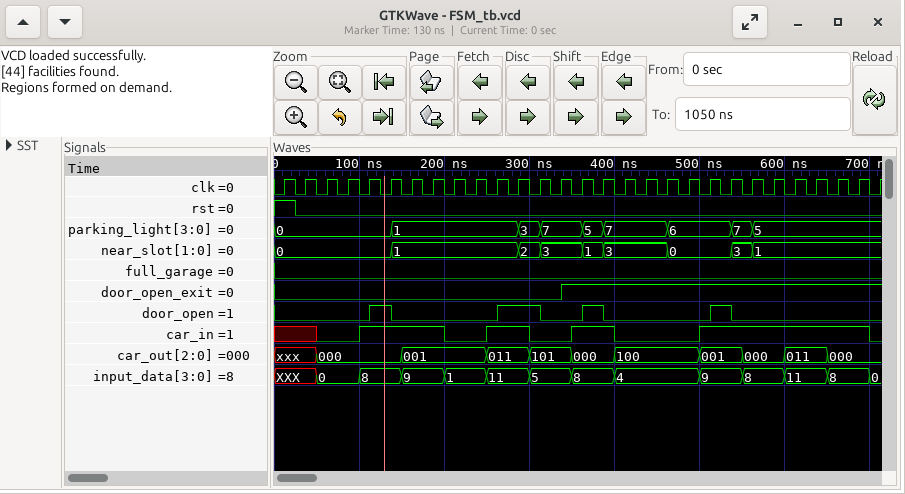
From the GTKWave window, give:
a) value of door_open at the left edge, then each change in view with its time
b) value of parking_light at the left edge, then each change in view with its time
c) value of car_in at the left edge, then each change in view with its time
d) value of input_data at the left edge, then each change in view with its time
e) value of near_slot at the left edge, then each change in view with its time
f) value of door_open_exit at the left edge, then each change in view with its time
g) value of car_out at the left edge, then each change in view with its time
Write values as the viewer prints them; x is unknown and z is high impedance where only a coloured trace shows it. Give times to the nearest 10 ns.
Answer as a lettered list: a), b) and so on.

a) 0, 1 at 110 ns, 0 at 140 ns, 1 at 260 ns, 0 at 310 ns, 1 at 360 ns, 0 at 390 ns, 1 at 510 ns, 0 at 540 ns
b) 0, 1 at 140 ns, 3 at 290 ns, 7 at 310 ns, 5 at 360 ns, 7 at 390 ns, 6 at 460 ns, 7 at 540 ns, 5 at 560 ns
c) x, 0 at 50 ns, 1 at 100 ns, 0 at 200 ns, 1 at 250 ns, 0 at 300 ns, 1 at 350 ns, 0 at 400 ns, 1 at 500 ns, 0 at 700 ns
d) XXX, 0 at 50 ns, 8 at 100 ns, 9 at 150 ns, 1 at 200 ns, 11 at 250 ns, 5 at 300 ns, 8 at 350 ns, 4 at 400 ns, 9 at 500 ns, 8 at 550 ns, 11 at 600 ns, 8 at 650 ns, 0 at 700 ns
e) 0, 1 at 140 ns, 2 at 290 ns, 3 at 310 ns, 1 at 360 ns, 3 at 390 ns, 0 at 460 ns, 3 at 540 ns, 1 at 560 ns
f) 0, 1 at 340 ns
g) xxx, 000 at 50 ns, 001 at 150 ns, 011 at 250 ns, 101 at 300 ns, 000 at 350 ns, 100 at 400 ns, 001 at 500 ns, 000 at 550 ns, 011 at 600 ns, 000 at 650 ns
